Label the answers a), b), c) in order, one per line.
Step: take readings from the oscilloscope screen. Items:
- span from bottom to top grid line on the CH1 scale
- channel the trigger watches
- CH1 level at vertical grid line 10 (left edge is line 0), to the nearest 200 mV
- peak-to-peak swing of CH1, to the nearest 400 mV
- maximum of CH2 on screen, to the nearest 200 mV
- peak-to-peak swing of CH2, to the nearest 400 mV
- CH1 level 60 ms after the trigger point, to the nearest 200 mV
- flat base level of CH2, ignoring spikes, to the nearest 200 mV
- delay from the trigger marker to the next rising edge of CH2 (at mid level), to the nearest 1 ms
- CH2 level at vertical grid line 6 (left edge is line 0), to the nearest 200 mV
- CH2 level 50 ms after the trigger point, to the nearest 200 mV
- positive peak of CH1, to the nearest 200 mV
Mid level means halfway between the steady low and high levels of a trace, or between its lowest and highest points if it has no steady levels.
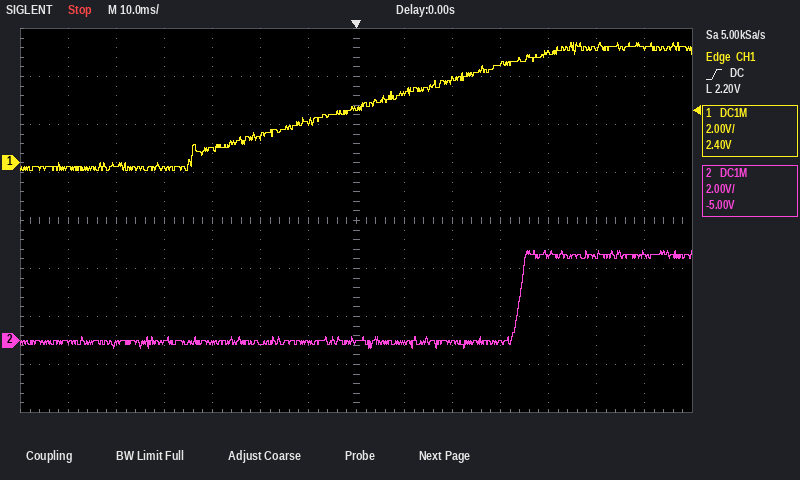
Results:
a) 16 V
b) CH1
c) 4.2 V
d) 5.2 V
e) 3.8 V
f) 4.0 V
g) 4.8 V
h) 0.0 V
i) 34 ms
j) 0.0 V
k) 3.6 V
l) 5.0 V
